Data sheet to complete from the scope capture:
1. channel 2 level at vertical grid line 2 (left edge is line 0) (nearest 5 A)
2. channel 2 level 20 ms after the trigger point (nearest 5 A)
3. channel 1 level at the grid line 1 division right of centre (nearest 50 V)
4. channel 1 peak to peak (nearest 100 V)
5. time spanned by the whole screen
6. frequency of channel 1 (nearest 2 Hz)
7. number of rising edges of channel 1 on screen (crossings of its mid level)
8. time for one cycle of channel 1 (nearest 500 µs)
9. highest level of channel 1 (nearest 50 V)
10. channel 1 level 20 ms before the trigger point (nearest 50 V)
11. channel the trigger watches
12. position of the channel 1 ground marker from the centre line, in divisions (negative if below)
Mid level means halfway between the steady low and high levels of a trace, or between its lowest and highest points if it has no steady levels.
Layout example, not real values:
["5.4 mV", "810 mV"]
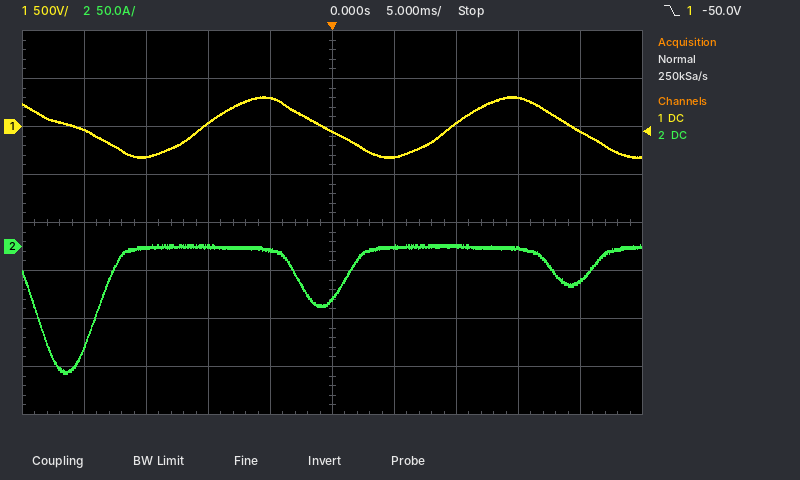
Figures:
["0 A", "-35 A", "-300 V", "600 V", "50 ms", "50 Hz", "2", "20.0 ms", "300 V", "-50 V", "channel 1", "+2.0 div"]
